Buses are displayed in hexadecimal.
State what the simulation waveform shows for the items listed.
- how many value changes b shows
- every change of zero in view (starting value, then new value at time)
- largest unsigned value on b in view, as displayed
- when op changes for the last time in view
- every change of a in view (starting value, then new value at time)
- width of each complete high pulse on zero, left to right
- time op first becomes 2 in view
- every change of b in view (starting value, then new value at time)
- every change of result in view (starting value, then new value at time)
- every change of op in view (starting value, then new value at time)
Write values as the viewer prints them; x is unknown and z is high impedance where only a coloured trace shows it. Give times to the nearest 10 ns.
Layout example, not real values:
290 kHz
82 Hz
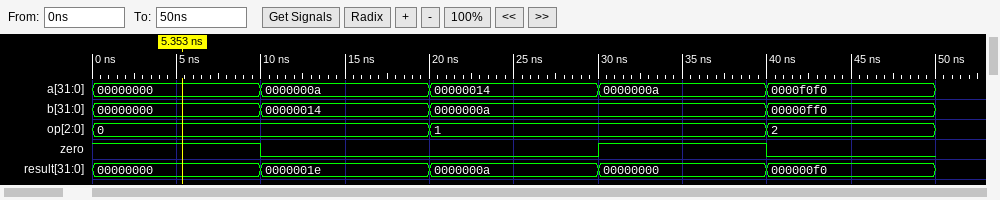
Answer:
3
1, 0 at 10 ns, 1 at 30 ns, 0 at 40 ns
00000ff0
40 ns
00000000, 0000000a at 10 ns, 00000014 at 20 ns, 0000000a at 30 ns, 0000f0f0 at 40 ns
10 ns
40 ns
00000000, 00000014 at 10 ns, 0000000a at 20 ns, 00000ff0 at 40 ns
00000000, 0000001e at 10 ns, 0000000a at 20 ns, 00000000 at 30 ns, 000000f0 at 40 ns
0, 1 at 20 ns, 2 at 40 ns
